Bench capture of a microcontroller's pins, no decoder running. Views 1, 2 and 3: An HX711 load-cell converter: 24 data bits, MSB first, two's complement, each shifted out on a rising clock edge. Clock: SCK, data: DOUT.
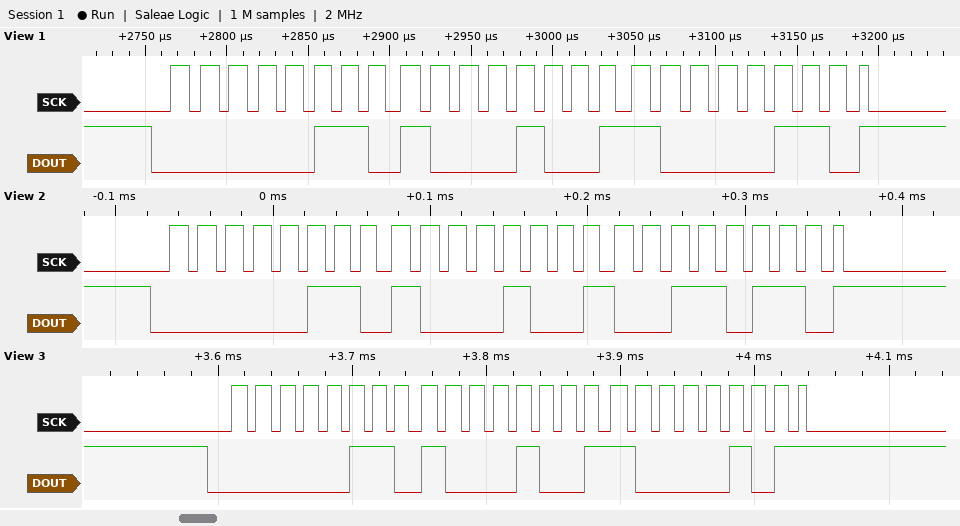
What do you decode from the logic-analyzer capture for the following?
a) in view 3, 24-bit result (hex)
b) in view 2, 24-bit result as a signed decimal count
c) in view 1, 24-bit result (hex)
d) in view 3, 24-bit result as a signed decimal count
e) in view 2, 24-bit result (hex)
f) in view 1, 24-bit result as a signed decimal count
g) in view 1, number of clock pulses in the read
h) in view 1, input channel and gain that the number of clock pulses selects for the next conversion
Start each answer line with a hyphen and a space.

- 0x068985
- 428342
- 0x068986
- 428421
- 0x068936
- 428422
- 25
- channel A, gain 128
